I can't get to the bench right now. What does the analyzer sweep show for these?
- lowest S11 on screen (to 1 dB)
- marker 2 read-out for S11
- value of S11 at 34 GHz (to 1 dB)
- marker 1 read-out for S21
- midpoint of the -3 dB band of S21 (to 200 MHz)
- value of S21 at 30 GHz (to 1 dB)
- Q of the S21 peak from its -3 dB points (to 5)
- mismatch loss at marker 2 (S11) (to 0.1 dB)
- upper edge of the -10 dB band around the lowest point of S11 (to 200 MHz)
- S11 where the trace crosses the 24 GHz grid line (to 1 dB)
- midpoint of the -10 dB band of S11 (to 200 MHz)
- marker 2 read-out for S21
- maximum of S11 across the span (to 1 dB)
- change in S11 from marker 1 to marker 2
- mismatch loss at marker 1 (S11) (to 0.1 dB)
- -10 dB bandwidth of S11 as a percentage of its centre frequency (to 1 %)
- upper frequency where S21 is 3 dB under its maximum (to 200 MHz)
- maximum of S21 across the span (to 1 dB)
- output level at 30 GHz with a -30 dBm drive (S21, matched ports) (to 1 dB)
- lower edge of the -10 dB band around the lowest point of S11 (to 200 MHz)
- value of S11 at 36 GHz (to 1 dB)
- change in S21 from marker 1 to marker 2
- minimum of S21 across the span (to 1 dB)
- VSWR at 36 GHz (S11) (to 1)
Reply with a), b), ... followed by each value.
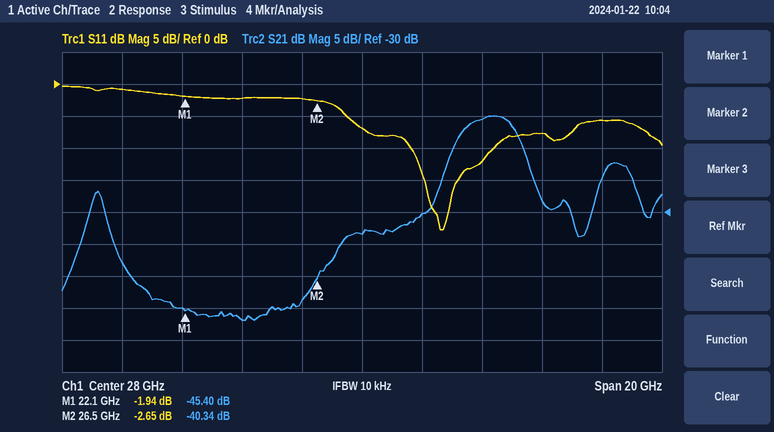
a) -23 dB
b) -2.65 dB
c) -8 dB
d) -45.40 dB
e) 32.2 GHz
f) -30 dB
g) 15
h) 3.4 dB
i) 32.4 GHz
j) -2 dB
k) 31.0 GHz
l) -40.34 dB
m) 0 dB
n) -0.71 dB
o) 4.4 dB
p) 9 %
q) 33.2 GHz
r) -15 dB
s) -60 dBm
t) 29.6 GHz
u) -6 dB
v) 5.06 dB
w) -47 dB
x) 3
